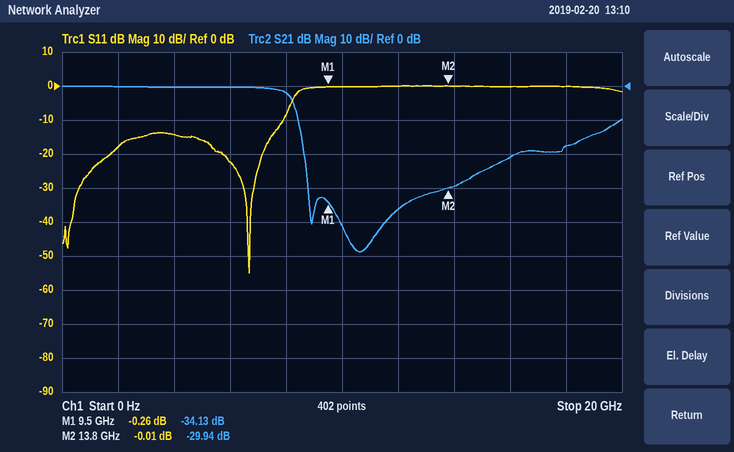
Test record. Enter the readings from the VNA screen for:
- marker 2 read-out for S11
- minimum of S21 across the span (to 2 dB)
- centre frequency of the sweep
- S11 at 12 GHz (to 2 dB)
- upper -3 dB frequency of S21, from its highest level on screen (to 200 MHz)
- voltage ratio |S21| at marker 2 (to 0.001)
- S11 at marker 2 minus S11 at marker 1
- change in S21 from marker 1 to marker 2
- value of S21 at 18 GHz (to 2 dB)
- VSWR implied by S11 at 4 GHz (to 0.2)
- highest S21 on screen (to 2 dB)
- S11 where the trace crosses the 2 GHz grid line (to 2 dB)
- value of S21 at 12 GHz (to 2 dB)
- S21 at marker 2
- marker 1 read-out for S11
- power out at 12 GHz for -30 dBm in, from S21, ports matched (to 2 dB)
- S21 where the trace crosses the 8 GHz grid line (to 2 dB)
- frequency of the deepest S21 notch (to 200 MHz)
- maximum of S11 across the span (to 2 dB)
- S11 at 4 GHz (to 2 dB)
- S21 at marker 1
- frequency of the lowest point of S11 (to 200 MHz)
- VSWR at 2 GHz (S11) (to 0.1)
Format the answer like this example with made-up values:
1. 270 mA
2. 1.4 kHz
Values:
1. -0.01 dB
2. -48 dB
3. 10 GHz
4. 0 dB
5. 8.2 GHz
6. 0.032
7. 0.25 dB
8. 4.19 dB
9. -18 dB
10. 1.4
11. 0 dB
12. -18 dB
13. -36 dB
14. -29.94 dB
15. -0.26 dB
16. -66 dBm
17. -2 dB
18. 10.6 GHz
19. 0 dB
20. -14 dB
21. -34.13 dB
22. 6.6 GHz
23. 1.3
